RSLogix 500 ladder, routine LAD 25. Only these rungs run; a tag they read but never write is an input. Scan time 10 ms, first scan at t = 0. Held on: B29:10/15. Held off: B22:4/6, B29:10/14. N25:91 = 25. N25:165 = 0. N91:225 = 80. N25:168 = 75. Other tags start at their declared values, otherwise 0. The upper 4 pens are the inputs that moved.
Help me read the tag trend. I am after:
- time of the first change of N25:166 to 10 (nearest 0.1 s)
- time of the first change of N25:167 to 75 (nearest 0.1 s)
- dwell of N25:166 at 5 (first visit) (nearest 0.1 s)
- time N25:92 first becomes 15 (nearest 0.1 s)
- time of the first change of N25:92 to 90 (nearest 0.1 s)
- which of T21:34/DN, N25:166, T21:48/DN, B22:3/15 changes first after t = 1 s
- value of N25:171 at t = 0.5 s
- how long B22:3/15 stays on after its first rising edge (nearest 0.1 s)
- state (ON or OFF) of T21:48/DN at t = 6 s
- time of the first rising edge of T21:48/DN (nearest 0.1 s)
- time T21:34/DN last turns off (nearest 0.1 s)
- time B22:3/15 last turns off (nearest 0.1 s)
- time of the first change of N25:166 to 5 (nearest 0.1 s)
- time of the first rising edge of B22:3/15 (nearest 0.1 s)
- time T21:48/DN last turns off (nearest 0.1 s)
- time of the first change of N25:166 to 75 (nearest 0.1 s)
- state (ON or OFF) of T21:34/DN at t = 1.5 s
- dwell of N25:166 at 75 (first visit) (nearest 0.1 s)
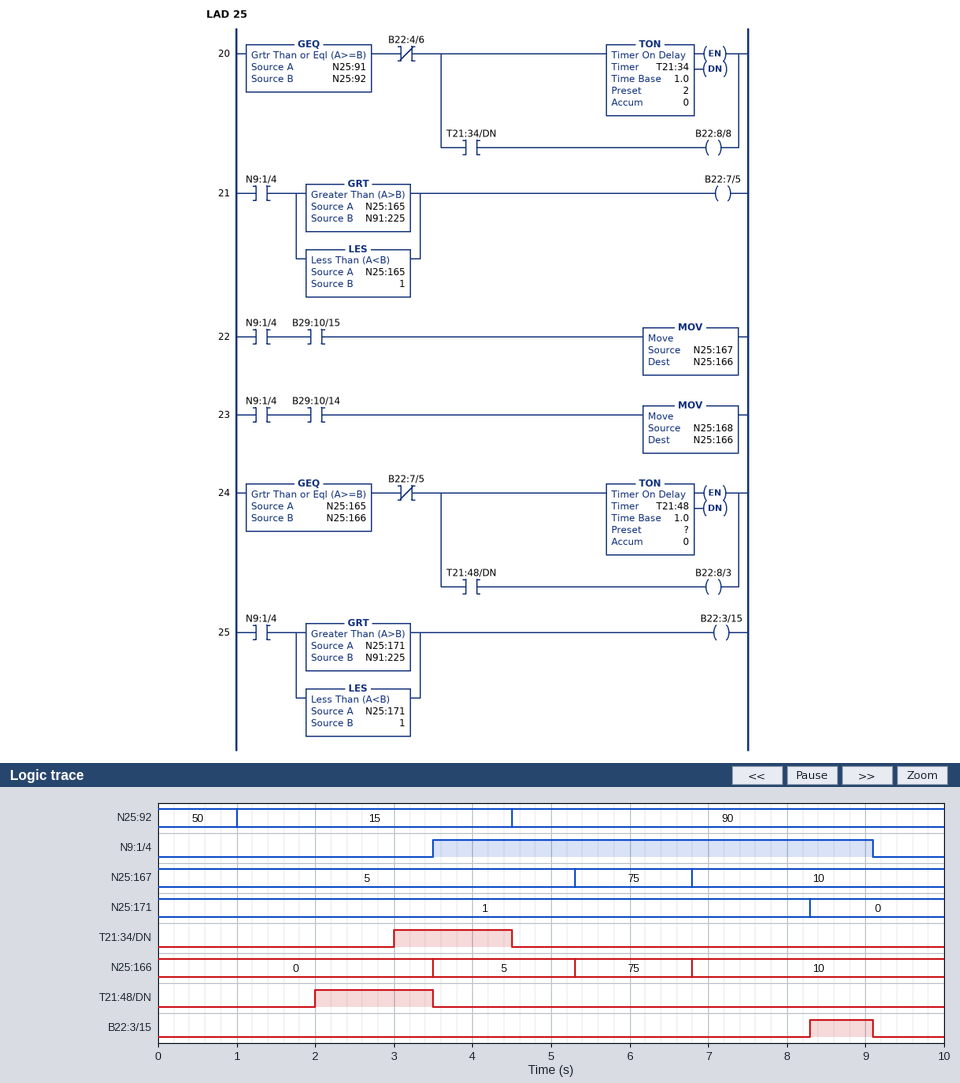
6.8 s
5.3 s
1.8 s
1.0 s
4.5 s
T21:48/DN
1
0.8 s
OFF
2.0 s
4.5 s
9.1 s
3.5 s
8.3 s
3.5 s
5.3 s
OFF
1.5 s
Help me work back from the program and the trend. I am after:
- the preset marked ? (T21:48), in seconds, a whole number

2 s
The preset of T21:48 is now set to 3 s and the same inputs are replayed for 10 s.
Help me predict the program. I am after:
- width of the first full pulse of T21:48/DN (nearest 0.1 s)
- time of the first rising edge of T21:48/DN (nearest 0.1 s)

0.5 s
3.0 s
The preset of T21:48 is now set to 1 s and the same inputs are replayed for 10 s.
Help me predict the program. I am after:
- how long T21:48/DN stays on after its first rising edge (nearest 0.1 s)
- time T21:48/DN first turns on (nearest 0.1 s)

2.5 s
1.0 s
